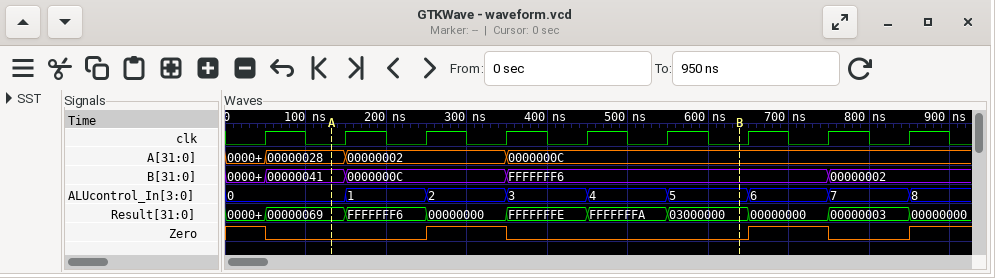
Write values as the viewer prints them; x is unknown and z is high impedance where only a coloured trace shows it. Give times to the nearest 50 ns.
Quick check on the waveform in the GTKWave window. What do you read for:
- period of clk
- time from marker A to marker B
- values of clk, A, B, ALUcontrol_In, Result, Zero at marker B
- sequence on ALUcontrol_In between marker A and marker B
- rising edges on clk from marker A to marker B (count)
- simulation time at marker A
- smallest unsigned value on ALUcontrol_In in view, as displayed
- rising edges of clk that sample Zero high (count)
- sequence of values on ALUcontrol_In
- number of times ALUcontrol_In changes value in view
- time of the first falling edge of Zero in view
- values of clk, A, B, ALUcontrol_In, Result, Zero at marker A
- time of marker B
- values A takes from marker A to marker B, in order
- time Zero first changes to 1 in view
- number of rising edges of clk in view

100 ns
500 ns
clk=0, A=0000000C, B=FFFFFFF6, ALUcontrol_In=5, Result=03000000, Zero=0
0, 1, 2, 3, 4, 5
5
150 ns
0
3
0, 1, 2, 3, 4, 5, 6, 7, 8
8
50 ns
clk=0, A=00000028, B=00000041, ALUcontrol_In=0, Result=00000069, Zero=0
650 ns
00000028, 00000002, 0000000C
250 ns
9
